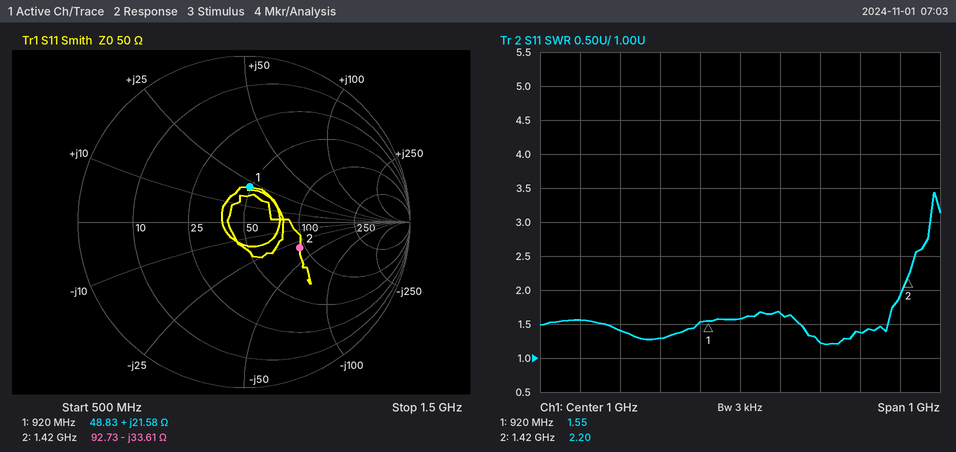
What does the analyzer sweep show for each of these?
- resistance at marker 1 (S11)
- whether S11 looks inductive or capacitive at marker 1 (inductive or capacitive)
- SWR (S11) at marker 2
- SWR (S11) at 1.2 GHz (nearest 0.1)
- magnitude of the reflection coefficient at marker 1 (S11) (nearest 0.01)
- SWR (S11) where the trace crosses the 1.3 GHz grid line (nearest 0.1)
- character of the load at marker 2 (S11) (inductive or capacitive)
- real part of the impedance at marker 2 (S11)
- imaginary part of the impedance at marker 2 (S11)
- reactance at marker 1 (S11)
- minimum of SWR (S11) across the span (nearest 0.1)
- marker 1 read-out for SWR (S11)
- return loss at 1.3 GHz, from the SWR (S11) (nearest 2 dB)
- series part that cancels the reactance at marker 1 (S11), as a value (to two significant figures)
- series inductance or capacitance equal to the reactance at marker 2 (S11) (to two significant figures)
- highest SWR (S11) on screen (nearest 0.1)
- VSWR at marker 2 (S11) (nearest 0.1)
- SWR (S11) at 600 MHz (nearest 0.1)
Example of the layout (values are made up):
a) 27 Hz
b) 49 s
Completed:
a) 48.83 Ω
b) inductive
c) 2.20
d) 1.2
e) 0.21
f) 1.4
g) capacitive
h) 92.73 Ω
i) -33.61 Ω
j) +21.58 Ω
k) 1.2
l) 1.55
m) 16 dB
n) 8.0 pF
o) 3.3 pF
p) 3.4
q) 2.2
r) 1.6
